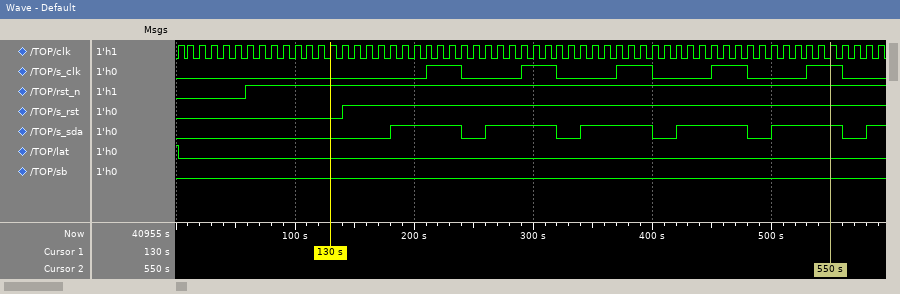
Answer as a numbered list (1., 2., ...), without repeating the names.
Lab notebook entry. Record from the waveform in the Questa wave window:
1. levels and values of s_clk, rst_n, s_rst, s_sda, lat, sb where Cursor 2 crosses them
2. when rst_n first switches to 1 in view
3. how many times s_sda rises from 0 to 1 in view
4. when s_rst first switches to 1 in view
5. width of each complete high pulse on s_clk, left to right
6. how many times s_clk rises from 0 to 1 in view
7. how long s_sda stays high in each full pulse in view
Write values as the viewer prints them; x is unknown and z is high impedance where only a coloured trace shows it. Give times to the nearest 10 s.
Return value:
1. s_clk=1, rst_n=1, s_rst=1, s_sda=1, lat=0, sb=0
2. 60 s
3. 6
4. 140 s
5. 30 s, 30 s, 30 s, 30 s, 30 s
6. 5
7. 60 s, 60 s, 60 s, 60 s, 60 s
